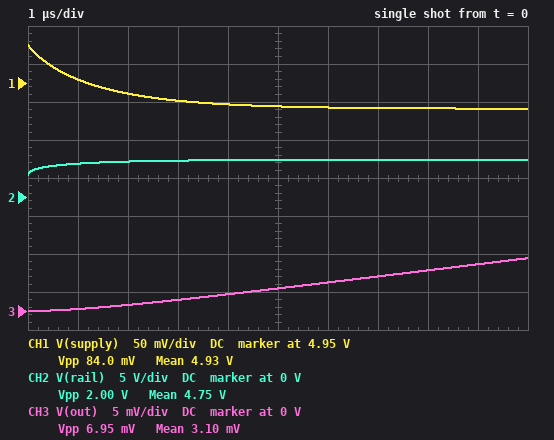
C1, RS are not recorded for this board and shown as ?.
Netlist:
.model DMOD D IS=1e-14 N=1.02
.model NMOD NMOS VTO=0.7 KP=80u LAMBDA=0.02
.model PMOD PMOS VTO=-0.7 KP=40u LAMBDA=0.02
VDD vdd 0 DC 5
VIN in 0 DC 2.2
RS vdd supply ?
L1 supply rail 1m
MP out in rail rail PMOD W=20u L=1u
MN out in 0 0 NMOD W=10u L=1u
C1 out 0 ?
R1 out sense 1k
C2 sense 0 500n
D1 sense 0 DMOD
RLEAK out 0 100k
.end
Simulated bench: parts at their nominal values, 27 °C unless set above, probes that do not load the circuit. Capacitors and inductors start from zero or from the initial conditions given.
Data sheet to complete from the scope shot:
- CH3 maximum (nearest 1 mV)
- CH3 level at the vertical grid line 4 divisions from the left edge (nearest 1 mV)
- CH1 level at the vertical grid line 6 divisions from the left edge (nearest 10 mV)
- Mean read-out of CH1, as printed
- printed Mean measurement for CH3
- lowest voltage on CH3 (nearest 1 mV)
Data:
7 mV
2 mV
4.92 V
4.93 V
3.10 mV
0 V
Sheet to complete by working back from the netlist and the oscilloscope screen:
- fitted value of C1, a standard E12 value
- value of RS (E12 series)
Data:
2.2 µF
47 Ω
